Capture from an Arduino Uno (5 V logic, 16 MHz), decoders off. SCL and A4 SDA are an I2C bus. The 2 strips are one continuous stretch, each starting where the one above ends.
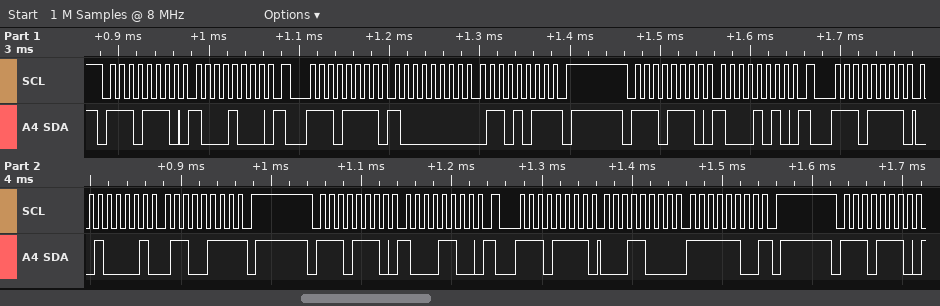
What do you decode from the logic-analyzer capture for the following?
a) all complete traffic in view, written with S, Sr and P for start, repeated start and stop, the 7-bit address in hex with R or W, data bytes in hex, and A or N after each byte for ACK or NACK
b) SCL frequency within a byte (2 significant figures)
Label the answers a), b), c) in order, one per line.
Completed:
a) S 77W A 88 A Sr 77R A 80 A 6B N P S 77W A 8A A Sr 77R A 21 A 67 N P S 77W A 8C A Sr 77R A 18 A FC N P S 77W A
b) 100 kHz
